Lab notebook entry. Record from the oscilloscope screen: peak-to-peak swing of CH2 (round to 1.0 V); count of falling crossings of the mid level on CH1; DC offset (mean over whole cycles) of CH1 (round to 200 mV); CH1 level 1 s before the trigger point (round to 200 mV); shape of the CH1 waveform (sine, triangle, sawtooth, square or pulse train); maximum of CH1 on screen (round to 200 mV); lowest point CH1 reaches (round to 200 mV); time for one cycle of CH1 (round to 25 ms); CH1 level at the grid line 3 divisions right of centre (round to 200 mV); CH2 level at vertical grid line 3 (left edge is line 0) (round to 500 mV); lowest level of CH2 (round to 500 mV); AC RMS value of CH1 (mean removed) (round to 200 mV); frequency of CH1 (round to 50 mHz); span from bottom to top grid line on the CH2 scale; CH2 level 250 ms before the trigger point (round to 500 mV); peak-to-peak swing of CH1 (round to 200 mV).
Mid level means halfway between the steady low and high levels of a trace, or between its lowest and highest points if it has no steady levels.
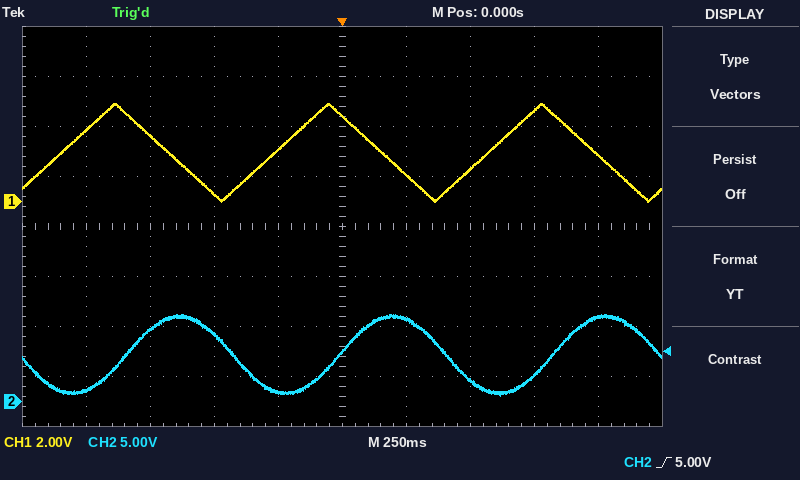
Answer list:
8.0 V
3
2.0 V
2.8 V
triangle
4.0 V
0.0 V
825 ms
3.6 V
6.5 V
500 mV
1.2 V
1.20 Hz
40 V
1.0 V
4.0 V
